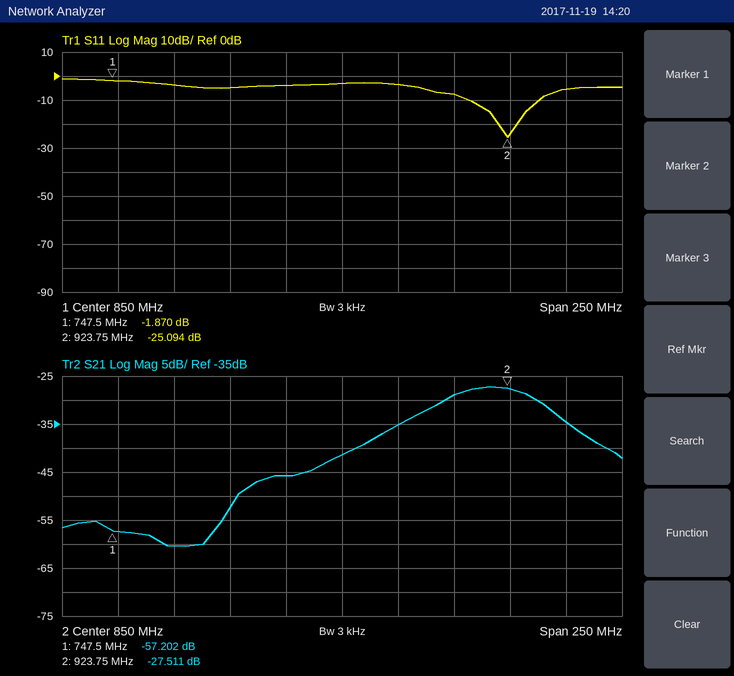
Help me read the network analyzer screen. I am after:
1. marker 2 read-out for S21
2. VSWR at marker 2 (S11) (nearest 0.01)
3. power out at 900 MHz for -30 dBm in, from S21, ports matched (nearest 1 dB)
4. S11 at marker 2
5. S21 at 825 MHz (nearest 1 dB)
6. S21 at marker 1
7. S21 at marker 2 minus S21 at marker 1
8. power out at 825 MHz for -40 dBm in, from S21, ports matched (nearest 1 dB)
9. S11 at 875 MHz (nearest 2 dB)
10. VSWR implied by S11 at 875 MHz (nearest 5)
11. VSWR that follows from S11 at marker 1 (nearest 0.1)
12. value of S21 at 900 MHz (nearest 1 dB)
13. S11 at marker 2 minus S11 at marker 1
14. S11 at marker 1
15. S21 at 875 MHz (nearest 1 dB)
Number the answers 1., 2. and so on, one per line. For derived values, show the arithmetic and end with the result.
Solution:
1. -27.511 dB
2. (1 + 0.0556)/(1 − 0.0556) ≈ 1.12
3. -30 dBm + (-29 dB) = -59 dBm
4. -25.094 dB
5. -46 dB
6. -57.202 dB
7. -27.511 − (-57.202) = 29.691 dB
8. -40 dBm + (-46 dB) = -86 dBm
9. -4 dB
10. |Γ| = 10^(-4/20) = 0.6310; VSWR = (1 + 0.6310)/(1 − 0.6310) ≈ 4.42, so 5 to the nearest 5
11. (1 + 0.8063)/(1 − 0.8063) ≈ 9.3
12. -29 dB
13. -25.094 − (-1.87) = -23.224 dB
14. -1.870 dB
15. -35 dB
